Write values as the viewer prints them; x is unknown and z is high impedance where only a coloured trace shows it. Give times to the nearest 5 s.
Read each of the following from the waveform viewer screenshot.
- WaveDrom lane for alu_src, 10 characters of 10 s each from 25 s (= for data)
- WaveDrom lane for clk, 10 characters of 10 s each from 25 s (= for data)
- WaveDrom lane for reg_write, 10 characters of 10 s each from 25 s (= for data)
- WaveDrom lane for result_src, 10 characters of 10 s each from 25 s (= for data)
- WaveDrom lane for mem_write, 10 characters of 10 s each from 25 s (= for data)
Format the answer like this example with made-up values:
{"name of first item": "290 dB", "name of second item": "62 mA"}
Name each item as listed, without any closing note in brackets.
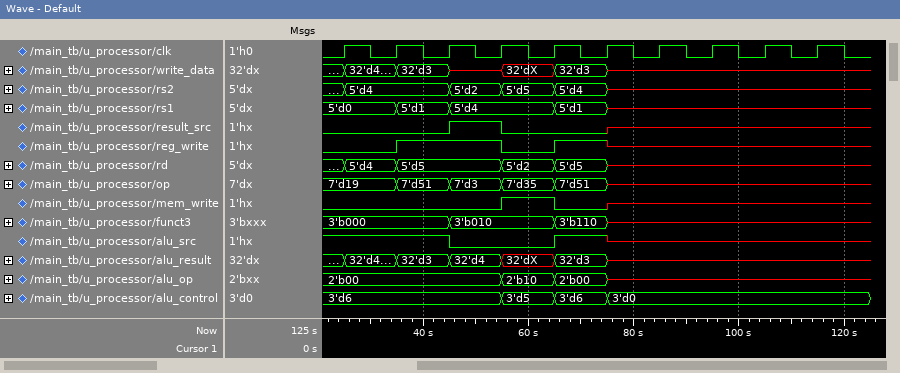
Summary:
{"WaveDrom lane for alu_src, 10 characters of 10 s each from 25 s": "{name: 'alu_src', wave: '1.0.1x....'}", "WaveDrom lane for clk, 10 characters of 10 s each from 25 s": "{name: 'clk', wave: 'p.........'}", "WaveDrom lane for reg_write, 10 characters of 10 s each from 25 s": "{name: 'reg_write', wave: '01.01x....'}", "WaveDrom lane for result_src, 10 characters of 10 s each from 25 s": "{name: 'result_src', wave: '0.10.x....'}", "WaveDrom lane for mem_write, 10 characters of 10 s each from 25 s": "{name: 'mem_write', wave: '0..10x....'}"}
